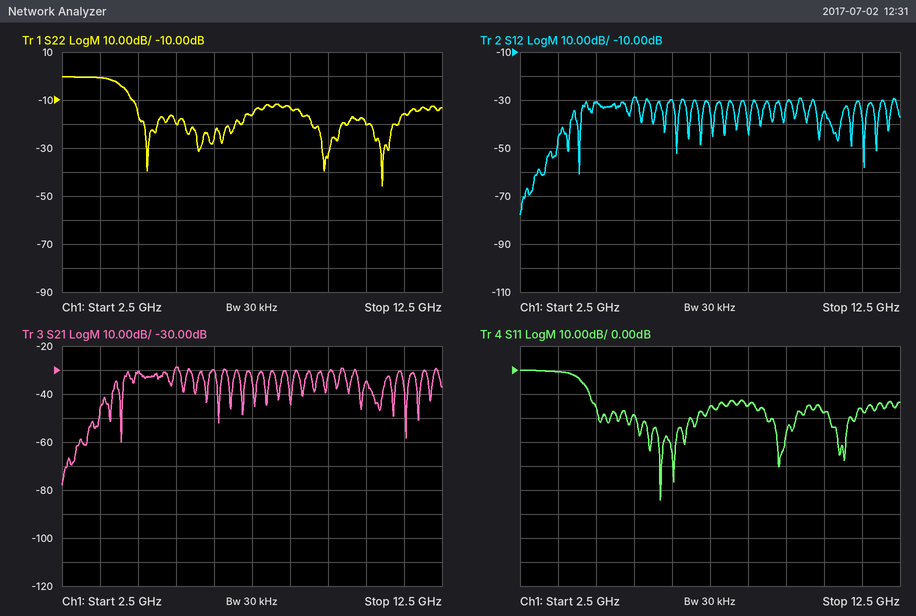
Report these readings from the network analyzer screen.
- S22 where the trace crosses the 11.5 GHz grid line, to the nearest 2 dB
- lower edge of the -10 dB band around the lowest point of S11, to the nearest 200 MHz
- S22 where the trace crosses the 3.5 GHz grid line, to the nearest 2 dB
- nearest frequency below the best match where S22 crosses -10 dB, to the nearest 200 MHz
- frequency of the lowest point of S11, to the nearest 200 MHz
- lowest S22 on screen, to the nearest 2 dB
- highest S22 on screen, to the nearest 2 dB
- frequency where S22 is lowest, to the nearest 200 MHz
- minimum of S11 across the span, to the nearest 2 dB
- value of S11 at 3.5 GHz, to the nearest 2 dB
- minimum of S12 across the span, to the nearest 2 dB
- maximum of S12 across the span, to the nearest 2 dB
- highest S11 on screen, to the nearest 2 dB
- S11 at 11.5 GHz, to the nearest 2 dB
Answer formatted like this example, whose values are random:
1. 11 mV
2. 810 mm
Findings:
1. -16 dB
2. 4.4 GHz
3. 0 dB
4. 4.4 GHz
5. 6.2 GHz
6. -46 dB
7. 0 dB
8. 11.0 GHz
9. -54 dB
10. 0 dB
11. -78 dB
12. -28 dB
13. 0 dB
14. -16 dB
